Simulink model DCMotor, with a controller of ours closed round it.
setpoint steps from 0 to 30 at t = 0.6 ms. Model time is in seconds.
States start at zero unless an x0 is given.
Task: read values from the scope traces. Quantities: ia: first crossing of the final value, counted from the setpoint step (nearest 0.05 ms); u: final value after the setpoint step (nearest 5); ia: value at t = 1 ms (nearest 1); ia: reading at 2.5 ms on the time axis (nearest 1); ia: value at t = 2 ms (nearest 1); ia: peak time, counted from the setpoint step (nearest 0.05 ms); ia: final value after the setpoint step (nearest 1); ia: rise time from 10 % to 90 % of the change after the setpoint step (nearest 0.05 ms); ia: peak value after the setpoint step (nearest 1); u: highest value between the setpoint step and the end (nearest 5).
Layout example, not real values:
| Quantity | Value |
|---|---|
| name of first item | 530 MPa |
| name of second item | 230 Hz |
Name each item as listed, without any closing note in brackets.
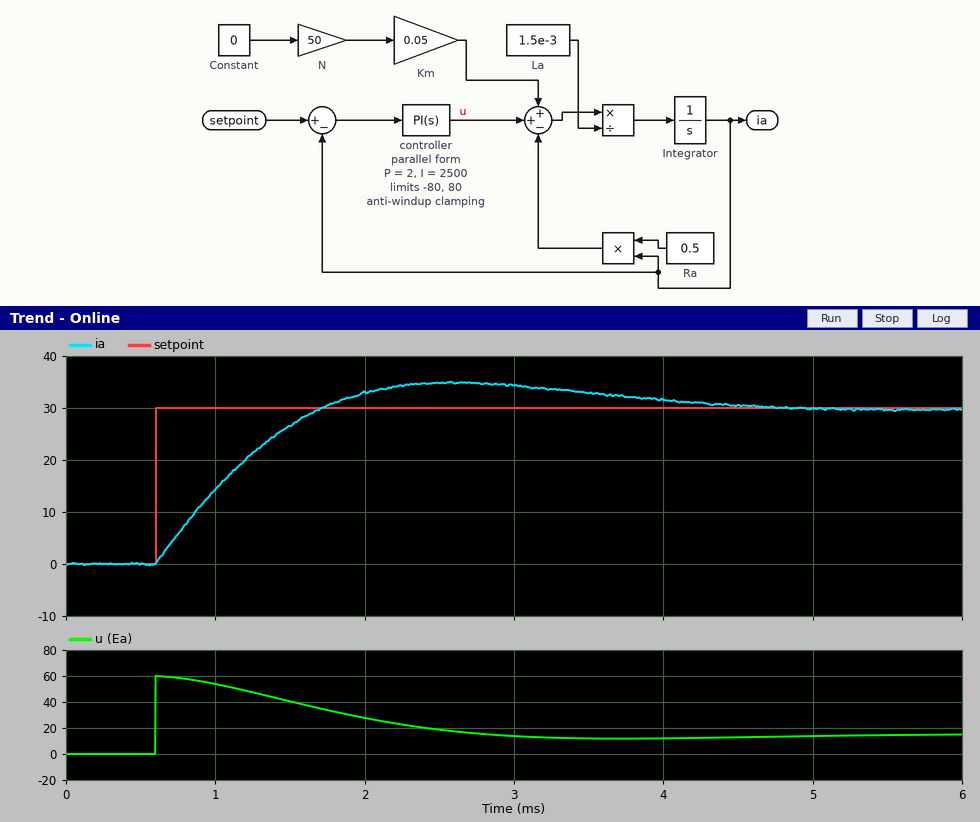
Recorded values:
| Quantity | Value |
|---|---|
| ia: first crossing of the final value, counted from the setpoint step | 1.10 ms |
| u: final value after the setpoint step | 15 |
| ia: value at t = 1 ms | 14 |
| ia: reading at 2.5 ms on the time axis | 35 |
| ia: value at t = 2 ms | 33 |
| ia: peak time, counted from the setpoint step | 2.00 ms |
| ia: final value after the setpoint step | 30 |
| ia: rise time from 10 % to 90 % of the change after the setpoint step | 0.85 ms |
| ia: peak value after the setpoint step | 35 |
| u: highest value between the setpoint step and the end | 60 |
